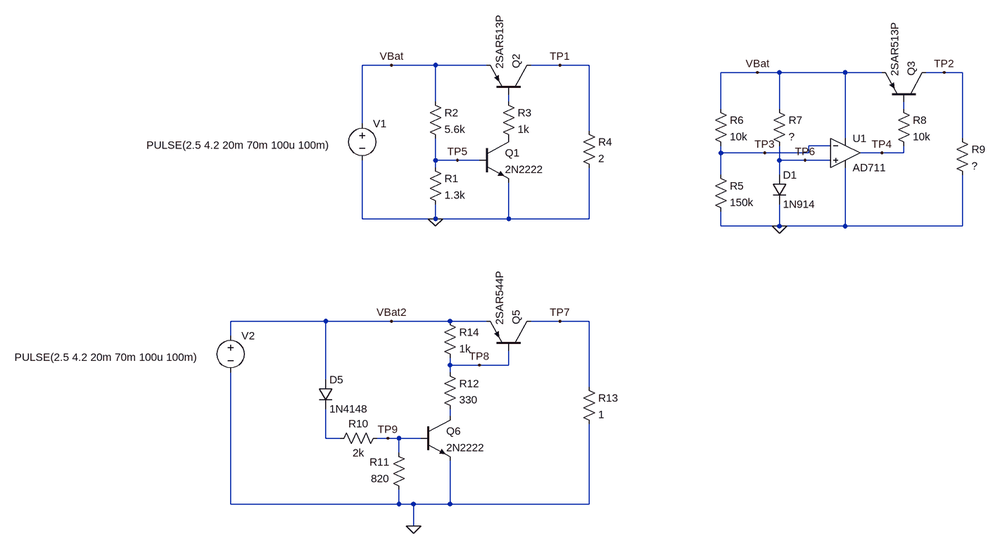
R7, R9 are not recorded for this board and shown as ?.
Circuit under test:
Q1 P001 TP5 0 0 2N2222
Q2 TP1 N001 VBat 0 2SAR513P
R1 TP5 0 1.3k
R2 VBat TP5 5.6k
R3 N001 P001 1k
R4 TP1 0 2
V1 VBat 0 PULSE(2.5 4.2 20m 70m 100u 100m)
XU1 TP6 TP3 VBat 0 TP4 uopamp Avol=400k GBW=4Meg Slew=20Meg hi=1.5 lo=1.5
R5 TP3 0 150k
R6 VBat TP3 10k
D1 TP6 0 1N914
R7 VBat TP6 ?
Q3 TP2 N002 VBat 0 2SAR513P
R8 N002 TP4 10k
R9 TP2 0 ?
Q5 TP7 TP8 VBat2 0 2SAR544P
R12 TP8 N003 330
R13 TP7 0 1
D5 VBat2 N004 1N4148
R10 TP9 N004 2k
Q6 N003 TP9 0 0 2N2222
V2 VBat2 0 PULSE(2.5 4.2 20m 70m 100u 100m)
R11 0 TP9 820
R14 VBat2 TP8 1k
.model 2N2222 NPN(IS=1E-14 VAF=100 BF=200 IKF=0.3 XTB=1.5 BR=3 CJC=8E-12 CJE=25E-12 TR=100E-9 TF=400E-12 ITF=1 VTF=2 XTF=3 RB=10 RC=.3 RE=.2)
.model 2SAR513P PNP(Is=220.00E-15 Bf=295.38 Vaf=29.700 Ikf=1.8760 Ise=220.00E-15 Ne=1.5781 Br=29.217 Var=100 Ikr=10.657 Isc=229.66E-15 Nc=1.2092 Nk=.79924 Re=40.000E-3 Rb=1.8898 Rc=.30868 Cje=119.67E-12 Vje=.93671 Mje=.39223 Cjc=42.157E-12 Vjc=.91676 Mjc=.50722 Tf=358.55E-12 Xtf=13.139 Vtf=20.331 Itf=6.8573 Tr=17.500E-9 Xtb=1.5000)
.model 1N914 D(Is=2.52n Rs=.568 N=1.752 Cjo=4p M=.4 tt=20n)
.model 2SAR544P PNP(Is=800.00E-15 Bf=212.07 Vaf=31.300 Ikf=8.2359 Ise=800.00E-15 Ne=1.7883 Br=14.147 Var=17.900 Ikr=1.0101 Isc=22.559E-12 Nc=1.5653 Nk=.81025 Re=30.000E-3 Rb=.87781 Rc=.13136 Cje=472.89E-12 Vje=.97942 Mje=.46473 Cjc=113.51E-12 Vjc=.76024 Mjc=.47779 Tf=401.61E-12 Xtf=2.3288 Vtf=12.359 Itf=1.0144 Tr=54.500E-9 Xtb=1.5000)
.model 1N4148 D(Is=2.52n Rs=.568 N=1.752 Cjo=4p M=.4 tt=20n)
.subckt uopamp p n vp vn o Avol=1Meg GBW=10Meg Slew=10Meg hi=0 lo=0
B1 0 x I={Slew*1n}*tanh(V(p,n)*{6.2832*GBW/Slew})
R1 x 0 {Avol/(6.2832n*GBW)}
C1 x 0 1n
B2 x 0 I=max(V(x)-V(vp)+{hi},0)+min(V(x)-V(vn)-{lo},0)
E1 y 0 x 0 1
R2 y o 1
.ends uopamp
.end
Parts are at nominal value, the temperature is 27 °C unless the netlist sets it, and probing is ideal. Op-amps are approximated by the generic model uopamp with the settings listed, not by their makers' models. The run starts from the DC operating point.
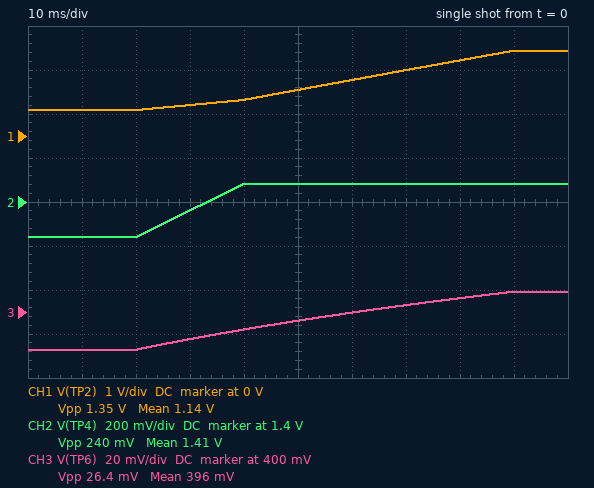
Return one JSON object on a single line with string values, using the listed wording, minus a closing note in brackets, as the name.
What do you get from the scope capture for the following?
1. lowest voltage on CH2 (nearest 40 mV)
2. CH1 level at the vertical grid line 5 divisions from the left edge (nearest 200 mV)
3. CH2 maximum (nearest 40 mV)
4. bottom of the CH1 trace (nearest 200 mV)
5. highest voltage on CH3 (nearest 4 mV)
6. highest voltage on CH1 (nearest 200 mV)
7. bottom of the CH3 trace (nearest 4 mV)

{"lowest voltage on CH2": "1.24 V", "CH1 level at the vertical grid line 5 divisions from the left edge": "1.0 V", "CH2 maximum": "1.48 V", "bottom of the CH1 trace": "600 mV", "highest voltage on CH3": "408 mV", "highest voltage on CH1": "2.0 V", "bottom of the CH3 trace": "384 mV"}
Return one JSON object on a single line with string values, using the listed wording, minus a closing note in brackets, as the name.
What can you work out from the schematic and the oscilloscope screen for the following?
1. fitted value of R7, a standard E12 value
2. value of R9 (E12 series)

{"fitted value of R7, a standard E12 value": "180 kΩ", "value of R9": "33 Ω"}
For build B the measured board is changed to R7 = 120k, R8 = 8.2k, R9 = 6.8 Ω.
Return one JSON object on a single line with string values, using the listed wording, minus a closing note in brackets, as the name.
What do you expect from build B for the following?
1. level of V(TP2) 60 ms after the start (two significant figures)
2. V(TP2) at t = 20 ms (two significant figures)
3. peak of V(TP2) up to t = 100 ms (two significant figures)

{"level of V(TP2) 60 ms after the start": "330 mV", "V(TP2) at t = 20 ms": "150 mV", "peak of V(TP2) up to t = 100 ms": "500 mV"}
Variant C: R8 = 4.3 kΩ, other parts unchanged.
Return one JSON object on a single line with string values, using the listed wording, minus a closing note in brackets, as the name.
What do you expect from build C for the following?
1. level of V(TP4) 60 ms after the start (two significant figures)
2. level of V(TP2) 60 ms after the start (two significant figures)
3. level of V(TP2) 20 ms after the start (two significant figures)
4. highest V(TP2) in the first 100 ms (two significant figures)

{"level of V(TP4) 60 ms after the start": "1.5 V", "level of V(TP2) 60 ms after the start": "2.7 V", "level of V(TP2) 20 ms after the start": "1.3 V", "highest V(TP2) in the first 100 ms": "3.9 V"}
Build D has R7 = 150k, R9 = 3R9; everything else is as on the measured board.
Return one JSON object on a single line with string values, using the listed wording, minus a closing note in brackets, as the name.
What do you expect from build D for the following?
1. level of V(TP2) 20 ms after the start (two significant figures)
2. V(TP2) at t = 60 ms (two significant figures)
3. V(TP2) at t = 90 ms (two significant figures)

{"level of V(TP2) 20 ms after the start": "71 mV", "V(TP2) at t = 60 ms": "160 mV", "V(TP2) at t = 90 ms": "240 mV"}
